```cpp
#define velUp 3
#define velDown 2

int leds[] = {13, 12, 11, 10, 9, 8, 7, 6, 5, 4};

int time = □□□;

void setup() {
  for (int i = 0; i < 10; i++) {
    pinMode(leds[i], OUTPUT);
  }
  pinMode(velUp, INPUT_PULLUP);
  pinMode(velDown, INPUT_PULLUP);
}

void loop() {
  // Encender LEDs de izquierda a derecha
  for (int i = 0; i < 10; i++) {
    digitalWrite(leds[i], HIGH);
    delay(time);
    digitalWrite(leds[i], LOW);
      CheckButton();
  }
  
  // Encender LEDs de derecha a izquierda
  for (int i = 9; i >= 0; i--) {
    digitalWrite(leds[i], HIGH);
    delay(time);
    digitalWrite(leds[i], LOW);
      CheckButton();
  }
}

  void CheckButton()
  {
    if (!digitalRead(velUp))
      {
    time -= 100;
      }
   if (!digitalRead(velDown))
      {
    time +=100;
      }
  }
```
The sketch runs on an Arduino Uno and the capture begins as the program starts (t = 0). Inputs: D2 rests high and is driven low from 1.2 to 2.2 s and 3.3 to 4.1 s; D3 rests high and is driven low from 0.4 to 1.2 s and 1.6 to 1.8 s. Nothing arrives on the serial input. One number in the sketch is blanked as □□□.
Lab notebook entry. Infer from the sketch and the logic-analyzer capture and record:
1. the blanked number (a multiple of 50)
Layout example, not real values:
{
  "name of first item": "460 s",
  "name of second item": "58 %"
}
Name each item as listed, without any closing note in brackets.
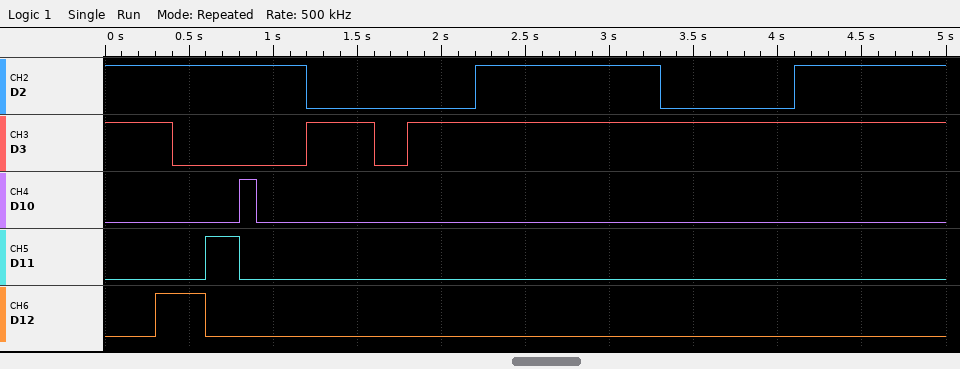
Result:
{
  "the blanked number": "300"
}
